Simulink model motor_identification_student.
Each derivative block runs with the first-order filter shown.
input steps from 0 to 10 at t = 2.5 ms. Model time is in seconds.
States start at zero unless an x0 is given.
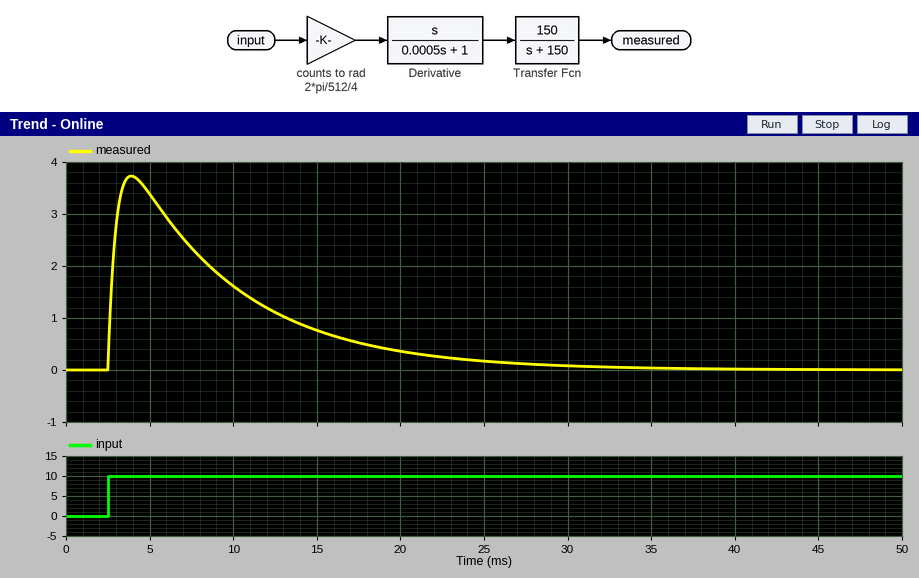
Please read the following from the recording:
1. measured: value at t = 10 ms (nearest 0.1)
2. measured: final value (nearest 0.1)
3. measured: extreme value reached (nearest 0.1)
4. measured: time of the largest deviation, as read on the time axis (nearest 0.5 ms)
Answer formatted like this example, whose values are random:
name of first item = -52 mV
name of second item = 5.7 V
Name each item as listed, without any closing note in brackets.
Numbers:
measured: value at t = 10 ms = 1.6
measured: final value = 0.0
measured: extreme value reached = 3.7
measured: time of the largest deviation, as read on the time axis = 4.0 ms
